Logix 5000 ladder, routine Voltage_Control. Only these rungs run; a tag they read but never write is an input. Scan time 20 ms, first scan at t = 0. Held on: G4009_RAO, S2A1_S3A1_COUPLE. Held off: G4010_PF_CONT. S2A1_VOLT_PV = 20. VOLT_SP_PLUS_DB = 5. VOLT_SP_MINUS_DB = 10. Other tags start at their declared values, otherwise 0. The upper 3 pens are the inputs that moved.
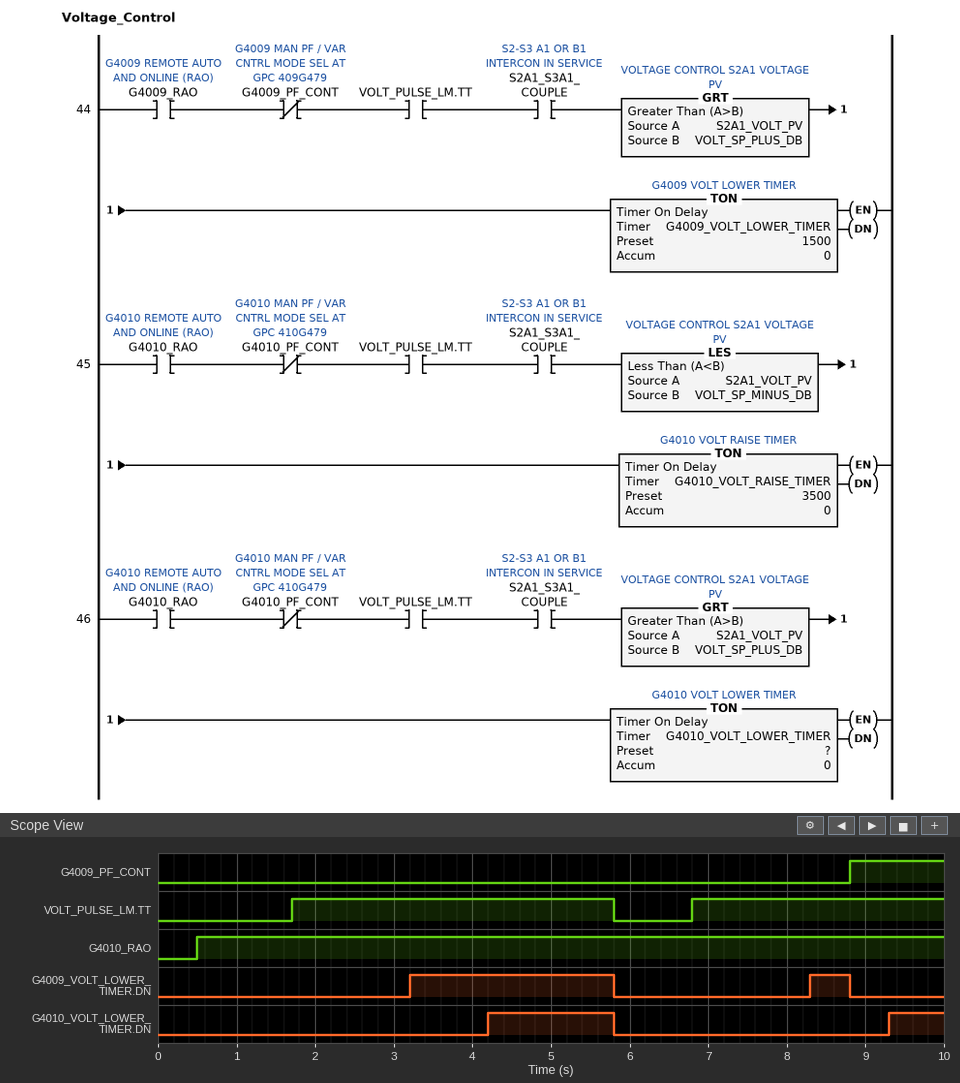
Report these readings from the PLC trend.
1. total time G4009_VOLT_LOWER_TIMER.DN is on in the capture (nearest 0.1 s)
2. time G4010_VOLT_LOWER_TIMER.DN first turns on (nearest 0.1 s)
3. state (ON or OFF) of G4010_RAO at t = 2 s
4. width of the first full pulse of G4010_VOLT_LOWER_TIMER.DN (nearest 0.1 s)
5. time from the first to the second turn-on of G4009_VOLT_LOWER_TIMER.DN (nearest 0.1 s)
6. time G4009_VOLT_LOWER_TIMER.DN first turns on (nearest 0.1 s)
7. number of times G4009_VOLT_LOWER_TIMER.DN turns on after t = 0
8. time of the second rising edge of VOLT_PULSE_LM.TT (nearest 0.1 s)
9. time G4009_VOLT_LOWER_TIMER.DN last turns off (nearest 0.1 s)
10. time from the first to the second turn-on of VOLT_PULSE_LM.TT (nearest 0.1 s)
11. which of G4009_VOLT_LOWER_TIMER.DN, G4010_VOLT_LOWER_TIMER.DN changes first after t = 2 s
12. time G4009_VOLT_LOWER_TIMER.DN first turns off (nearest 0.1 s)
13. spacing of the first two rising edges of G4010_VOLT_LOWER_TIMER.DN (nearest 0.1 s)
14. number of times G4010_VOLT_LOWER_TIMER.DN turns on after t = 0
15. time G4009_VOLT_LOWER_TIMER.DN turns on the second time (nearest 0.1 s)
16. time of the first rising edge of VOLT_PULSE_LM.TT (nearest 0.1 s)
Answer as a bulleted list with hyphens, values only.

- 3.1 s
- 4.2 s
- ON
- 1.6 s
- 5.1 s
- 3.2 s
- 2
- 6.8 s
- 8.8 s
- 5.1 s
- G4009_VOLT_LOWER_TIMER.DN
- 5.8 s
- 5.1 s
- 2
- 8.3 s
- 1.7 s
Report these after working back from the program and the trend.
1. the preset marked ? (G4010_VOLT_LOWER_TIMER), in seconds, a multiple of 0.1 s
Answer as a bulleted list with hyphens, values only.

- 2.5 s
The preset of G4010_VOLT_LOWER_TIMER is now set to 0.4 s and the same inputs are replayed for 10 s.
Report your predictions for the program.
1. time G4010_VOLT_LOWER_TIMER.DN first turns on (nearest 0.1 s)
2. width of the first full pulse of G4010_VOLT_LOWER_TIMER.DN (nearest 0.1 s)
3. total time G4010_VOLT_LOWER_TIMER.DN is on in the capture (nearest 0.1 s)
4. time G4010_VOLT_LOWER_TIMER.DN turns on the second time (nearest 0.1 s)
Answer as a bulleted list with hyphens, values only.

- 2.1 s
- 3.7 s
- 6.5 s
- 7.2 s
